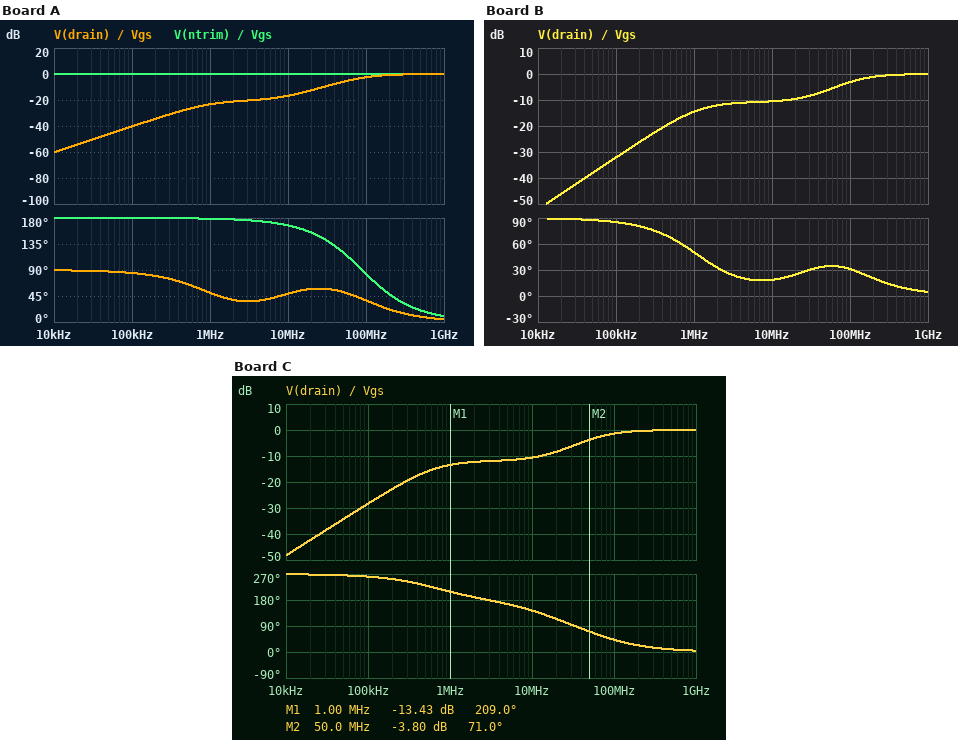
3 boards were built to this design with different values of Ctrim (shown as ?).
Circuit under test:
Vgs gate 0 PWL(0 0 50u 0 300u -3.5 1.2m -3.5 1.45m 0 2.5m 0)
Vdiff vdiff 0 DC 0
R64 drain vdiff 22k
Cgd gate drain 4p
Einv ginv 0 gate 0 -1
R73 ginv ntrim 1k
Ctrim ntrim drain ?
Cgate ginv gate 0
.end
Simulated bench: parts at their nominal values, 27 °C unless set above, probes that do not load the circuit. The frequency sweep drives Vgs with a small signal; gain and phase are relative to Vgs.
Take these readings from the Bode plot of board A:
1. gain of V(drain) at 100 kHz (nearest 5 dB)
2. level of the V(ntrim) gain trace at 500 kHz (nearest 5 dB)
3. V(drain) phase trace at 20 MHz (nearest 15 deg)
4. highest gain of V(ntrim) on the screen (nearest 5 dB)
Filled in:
-40 dB
0 dB
60 deg
0 dB
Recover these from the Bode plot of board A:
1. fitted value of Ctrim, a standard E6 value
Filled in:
3.3 pF
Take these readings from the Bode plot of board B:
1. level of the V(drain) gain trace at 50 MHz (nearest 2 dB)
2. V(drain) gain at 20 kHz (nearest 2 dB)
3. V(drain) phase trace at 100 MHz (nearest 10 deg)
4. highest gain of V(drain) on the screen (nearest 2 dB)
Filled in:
-6 dB
-46 dB
30 deg
0 dB
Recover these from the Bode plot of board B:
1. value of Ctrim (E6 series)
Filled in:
2.2 pF
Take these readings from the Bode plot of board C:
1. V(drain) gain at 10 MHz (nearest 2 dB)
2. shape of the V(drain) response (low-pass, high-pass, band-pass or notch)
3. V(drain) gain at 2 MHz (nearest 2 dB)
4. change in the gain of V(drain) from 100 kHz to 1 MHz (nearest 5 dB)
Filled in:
-10 dB
high-pass
-12 dB
15 dB
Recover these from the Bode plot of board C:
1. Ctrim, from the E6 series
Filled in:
6.8 pF
